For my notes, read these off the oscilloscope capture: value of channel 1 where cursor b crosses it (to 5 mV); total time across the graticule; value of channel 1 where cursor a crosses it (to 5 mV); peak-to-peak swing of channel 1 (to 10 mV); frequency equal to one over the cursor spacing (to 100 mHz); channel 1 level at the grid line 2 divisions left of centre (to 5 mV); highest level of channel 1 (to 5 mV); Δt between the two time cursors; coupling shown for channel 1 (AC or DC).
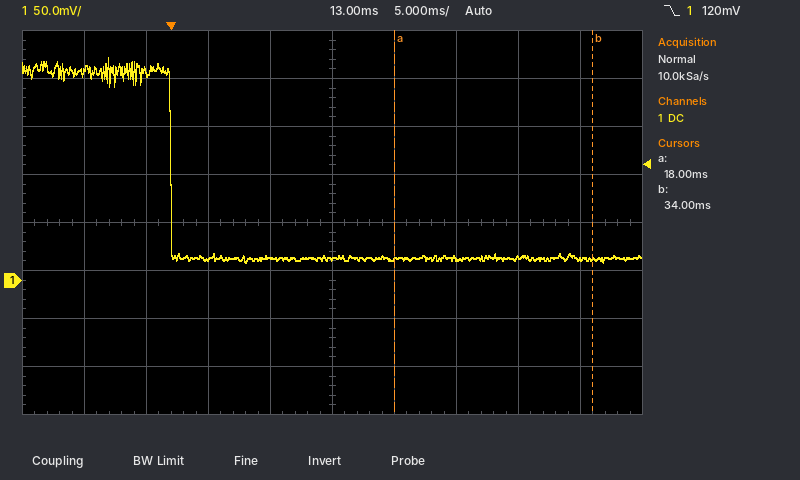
20 mV
50 ms
20 mV
210 mV
62.5 Hz
20 mV
230 mV
16.0 ms
DC
